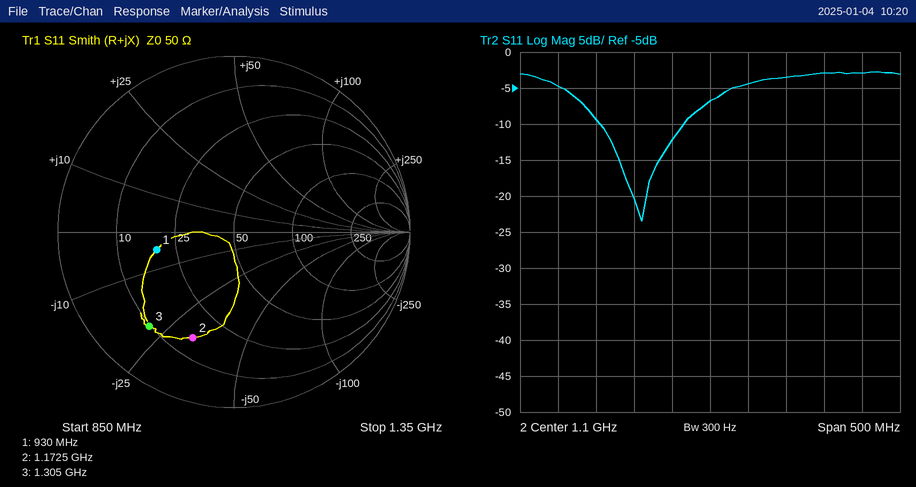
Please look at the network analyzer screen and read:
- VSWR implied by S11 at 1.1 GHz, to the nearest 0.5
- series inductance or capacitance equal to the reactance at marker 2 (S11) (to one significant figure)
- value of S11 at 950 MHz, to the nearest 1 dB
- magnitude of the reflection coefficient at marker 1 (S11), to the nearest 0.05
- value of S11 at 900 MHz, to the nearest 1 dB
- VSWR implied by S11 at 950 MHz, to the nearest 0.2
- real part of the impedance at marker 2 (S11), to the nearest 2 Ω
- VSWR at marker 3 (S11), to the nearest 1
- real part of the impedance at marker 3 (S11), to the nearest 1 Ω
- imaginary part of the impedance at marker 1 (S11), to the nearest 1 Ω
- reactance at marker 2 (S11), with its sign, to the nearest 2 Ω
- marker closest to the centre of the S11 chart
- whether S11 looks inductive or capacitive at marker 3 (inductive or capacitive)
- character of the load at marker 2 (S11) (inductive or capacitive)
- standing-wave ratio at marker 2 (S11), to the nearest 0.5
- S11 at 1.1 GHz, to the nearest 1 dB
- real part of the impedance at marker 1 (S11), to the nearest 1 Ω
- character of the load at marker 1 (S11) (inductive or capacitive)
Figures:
2.5
4 pF
-9 dB
0.45
-5 dB
2.0
16 Ω
6
10 Ω
-5 Ω
-32 Ω
marker 1
capacitive
capacitive
4.5
-7 dB
19 Ω
capacitive
